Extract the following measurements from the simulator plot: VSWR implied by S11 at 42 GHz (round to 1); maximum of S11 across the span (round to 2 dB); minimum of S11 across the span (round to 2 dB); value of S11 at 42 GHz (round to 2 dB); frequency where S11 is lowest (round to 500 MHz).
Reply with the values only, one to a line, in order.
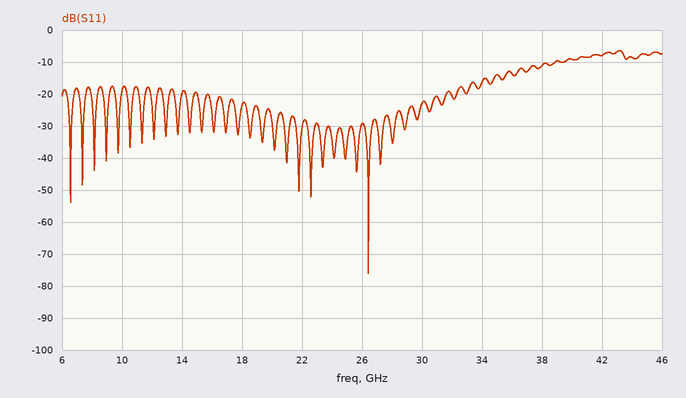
2
-6 dB
-76 dB
-8 dB
26.5 GHz
